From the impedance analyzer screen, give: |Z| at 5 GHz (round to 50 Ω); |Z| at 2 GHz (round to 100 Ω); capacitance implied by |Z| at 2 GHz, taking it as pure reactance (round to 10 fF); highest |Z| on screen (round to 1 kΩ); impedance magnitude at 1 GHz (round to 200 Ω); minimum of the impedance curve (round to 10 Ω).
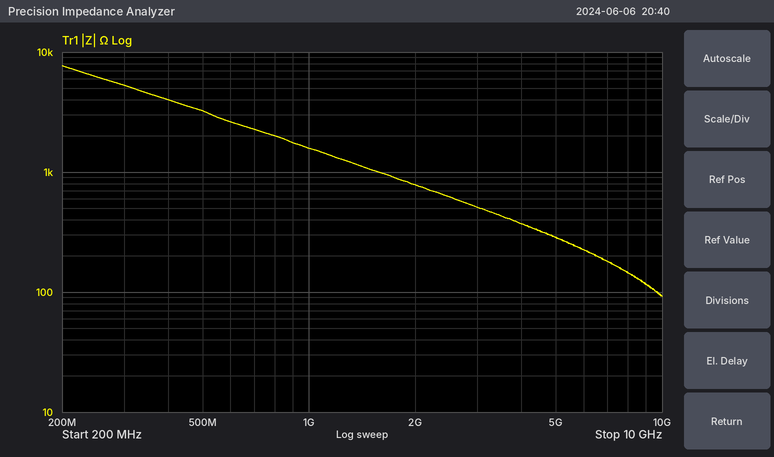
300 Ω
800 Ω
100 fF
8 kΩ
1.6 kΩ
90 Ω
